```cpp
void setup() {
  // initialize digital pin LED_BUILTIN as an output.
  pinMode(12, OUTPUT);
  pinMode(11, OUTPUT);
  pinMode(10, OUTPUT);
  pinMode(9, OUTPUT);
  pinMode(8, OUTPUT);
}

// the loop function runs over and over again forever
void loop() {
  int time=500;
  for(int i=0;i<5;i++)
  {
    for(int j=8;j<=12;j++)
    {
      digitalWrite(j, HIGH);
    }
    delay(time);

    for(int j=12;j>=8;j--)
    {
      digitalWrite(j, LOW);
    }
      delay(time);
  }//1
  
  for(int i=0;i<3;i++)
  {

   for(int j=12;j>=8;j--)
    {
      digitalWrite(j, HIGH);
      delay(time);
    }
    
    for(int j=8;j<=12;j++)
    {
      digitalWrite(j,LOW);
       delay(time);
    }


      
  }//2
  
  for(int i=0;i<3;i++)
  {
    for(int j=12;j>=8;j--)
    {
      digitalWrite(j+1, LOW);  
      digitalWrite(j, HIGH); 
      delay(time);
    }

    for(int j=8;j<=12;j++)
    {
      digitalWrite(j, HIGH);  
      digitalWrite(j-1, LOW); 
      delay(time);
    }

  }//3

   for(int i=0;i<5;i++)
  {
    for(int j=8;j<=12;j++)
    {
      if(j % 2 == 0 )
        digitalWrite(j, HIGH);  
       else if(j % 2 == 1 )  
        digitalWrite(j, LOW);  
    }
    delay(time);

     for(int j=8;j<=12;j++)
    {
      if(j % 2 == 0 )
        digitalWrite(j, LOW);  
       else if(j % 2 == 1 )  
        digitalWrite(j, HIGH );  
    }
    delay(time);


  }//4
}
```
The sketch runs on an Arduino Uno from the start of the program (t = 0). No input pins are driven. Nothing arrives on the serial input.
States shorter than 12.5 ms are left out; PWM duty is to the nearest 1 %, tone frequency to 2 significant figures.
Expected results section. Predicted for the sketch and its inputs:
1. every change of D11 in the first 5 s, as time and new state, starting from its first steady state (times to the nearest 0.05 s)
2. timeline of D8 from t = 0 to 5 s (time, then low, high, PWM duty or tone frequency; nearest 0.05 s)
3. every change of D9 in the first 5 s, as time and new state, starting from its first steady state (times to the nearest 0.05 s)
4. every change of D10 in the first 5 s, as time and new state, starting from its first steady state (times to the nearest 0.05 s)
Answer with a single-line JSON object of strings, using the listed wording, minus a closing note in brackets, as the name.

{"every change of D11 in the first 5 s, as time and new state, starting from its first steady state": "0 s high; 0.5 s low; 1 s high; 1.5 s low; 2 s high; 2.5 s low; 3 s high; 3.5 s low; 4 s high; 4.5 s low", "timeline of D8 from t = 0 to 5 s": "0 s high; 0.5 s low; 1 s high; 1.5 s low; 2 s high; 2.5 s low; 3 s high; 3.5 s low; 4 s high; 4.5 s low", "every change of D9 in the first 5 s, as time and new state, starting from its first steady state": "0 s high; 0.5 s low; 1 s high; 1.5 s low; 2 s high; 2.5 s low; 3 s high; 3.5 s low; 4 s high; 4.5 s low", "every change of D10 in the first 5 s, as time and new state, starting from its first steady state": "0 s high; 0.5 s low; 1 s high; 1.5 s low; 2 s high; 2.5 s low; 3 s high; 3.5 s low; 4 s high; 4.5 s low"}
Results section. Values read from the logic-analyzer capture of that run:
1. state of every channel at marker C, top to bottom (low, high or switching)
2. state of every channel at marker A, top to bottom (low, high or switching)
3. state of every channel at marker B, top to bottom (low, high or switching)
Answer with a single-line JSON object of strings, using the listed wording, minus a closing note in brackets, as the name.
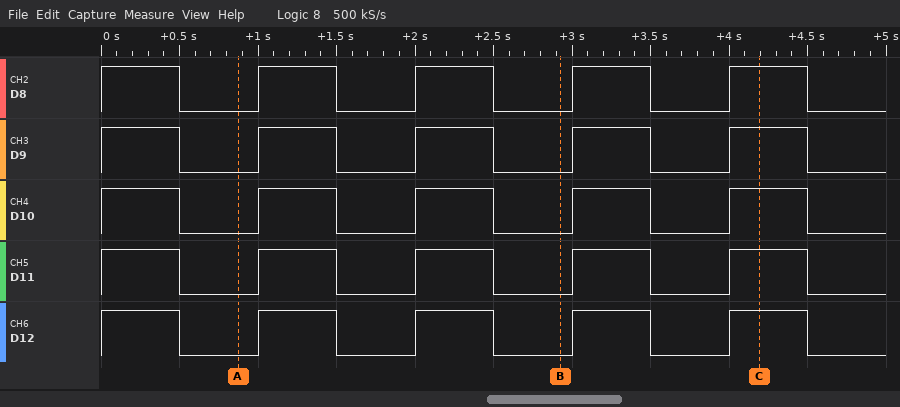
{"state of every channel at marker C, top to bottom": "D8 high, D9 high, D10 high, D11 high, D12 high", "state of every channel at marker A, top to bottom": "D8 low, D9 low, D10 low, D11 low, D12 low", "state of every channel at marker B, top to bottom": "D8 low, D9 low, D10 low, D11 low, D12 low"}
